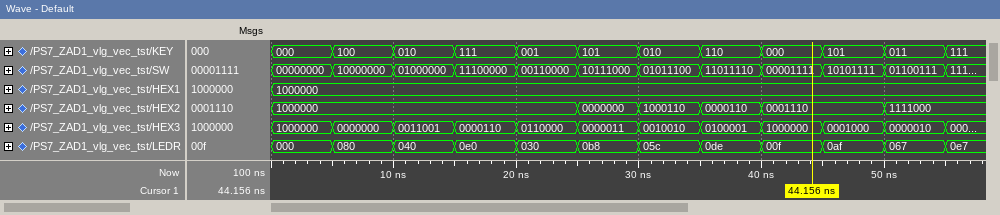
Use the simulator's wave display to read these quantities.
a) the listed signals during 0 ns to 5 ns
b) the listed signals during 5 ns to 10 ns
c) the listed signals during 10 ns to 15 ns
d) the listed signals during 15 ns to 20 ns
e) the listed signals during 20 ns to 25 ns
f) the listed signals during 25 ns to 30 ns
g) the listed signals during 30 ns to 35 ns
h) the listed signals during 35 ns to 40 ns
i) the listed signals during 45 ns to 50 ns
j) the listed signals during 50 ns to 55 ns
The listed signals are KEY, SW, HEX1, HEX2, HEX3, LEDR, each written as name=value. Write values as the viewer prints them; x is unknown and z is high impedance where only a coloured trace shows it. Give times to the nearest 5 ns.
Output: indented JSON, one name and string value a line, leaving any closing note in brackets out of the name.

{
  "the listed signals during 0 ns to 5 ns": "KEY=000, SW=00000000, HEX1=1000000, HEX2=1000000, HEX3=1000000, LEDR=000",
  "the listed signals during 5 ns to 10 ns": "KEY=100, SW=10000000, HEX1=1000000, HEX2=1000000, HEX3=0000000, LEDR=080",
  "the listed signals during 10 ns to 15 ns": "KEY=010, SW=01000000, HEX1=1000000, HEX2=1000000, HEX3=0011001, LEDR=040",
  "the listed signals during 15 ns to 20 ns": "KEY=111, SW=11100000, HEX1=1000000, HEX2=1000000, HEX3=0000110, LEDR=0e0",
  "the listed signals during 20 ns to 25 ns": "KEY=001, SW=00110000, HEX1=1000000, HEX2=1000000, HEX3=0110000, LEDR=030",
  "the listed signals during 25 ns to 30 ns": "KEY=101, SW=10111000, HEX1=1000000, HEX2=0000000, HEX3=0000011, LEDR=0b8",
  "the listed signals during 30 ns to 35 ns": "KEY=010, SW=01011100, HEX1=1000000, HEX2=1000110, HEX3=0010010, LEDR=05c",
  "the listed signals during 35 ns to 40 ns": "KEY=110, SW=11011110, HEX1=1000000, HEX2=0000110, HEX3=0100001, LEDR=0de",
  "the listed signals during 45 ns to 50 ns": "KEY=101, SW=10101111, HEX1=1000000, HEX2=0001110, HEX3=0001000, LEDR=0af",
  "the listed signals during 50 ns to 55 ns": "KEY=011, SW=01100111, HEX1=1000000, HEX2=1111000, HEX3=0000010, LEDR=067"
}
